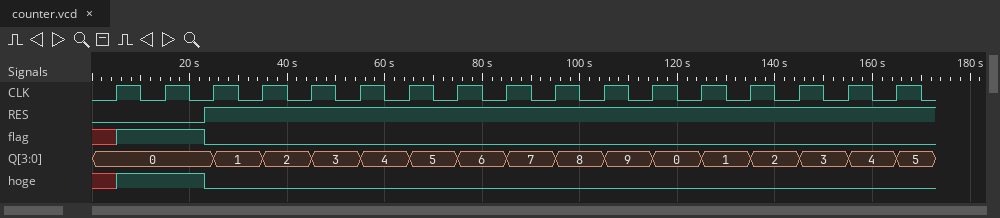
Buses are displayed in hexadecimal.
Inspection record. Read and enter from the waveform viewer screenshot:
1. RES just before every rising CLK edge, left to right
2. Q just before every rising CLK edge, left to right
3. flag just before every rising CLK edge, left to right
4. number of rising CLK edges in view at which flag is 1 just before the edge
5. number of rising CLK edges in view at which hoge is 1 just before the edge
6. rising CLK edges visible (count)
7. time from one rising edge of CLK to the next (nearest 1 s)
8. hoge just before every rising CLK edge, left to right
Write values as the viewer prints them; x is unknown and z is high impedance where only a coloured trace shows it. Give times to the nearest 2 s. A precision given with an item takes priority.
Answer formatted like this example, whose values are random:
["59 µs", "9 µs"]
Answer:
["0 0 1 1 1 1 1 1 1 1 1 1 1 1 1 1 1", "0, 0, 0, 1, 2, 3, 4, 5, 6, 7, 8, 9, 0, 1, 2, 3, 4", "x 1 0 0 0 0 0 0 0 0 0 0 0 0 0 0 0", "1", "1", "17", "10 s", "x 1 0 0 0 0 0 0 0 0 0 0 0 0 0 0 0"]
